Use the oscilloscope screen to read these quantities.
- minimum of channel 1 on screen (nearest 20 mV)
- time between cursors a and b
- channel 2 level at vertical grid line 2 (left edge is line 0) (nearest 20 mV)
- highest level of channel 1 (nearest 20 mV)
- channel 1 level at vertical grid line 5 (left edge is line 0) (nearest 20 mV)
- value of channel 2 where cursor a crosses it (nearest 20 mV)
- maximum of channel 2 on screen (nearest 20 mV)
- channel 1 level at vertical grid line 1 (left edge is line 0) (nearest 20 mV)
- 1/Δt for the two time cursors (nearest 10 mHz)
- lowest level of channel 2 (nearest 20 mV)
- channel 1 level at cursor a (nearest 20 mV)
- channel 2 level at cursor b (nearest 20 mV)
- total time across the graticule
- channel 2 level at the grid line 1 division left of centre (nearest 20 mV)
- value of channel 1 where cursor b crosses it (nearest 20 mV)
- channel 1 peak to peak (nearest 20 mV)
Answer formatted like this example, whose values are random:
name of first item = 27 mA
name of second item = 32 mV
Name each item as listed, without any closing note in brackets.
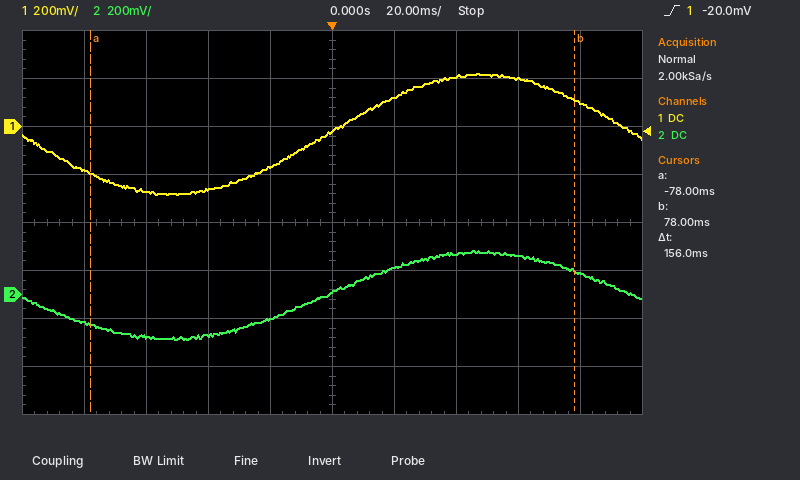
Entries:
minimum of channel 1 on screen = -280 mV
time between cursors a and b = 156 ms
channel 2 level at vertical grid line 2 (left edge is line 0) = -180 mV
highest level of channel 1 = 220 mV
channel 1 level at vertical grid line 5 (left edge is line 0) = -20 mV
value of channel 2 where cursor a crosses it = -120 mV
maximum of channel 2 on screen = 180 mV
channel 1 level at vertical grid line 1 (left edge is line 0) = -180 mV
1/Δt for the two time cursors = 6.41 Hz
lowest level of channel 2 = -180 mV
channel 1 level at cursor a = -200 mV
channel 2 level at cursor b = 100 mV
total time across the graticule = 200 ms
channel 2 level at the grid line 1 division left of centre = -100 mV
value of channel 1 where cursor b crosses it = 120 mV
channel 1 peak to peak = 500 mV
